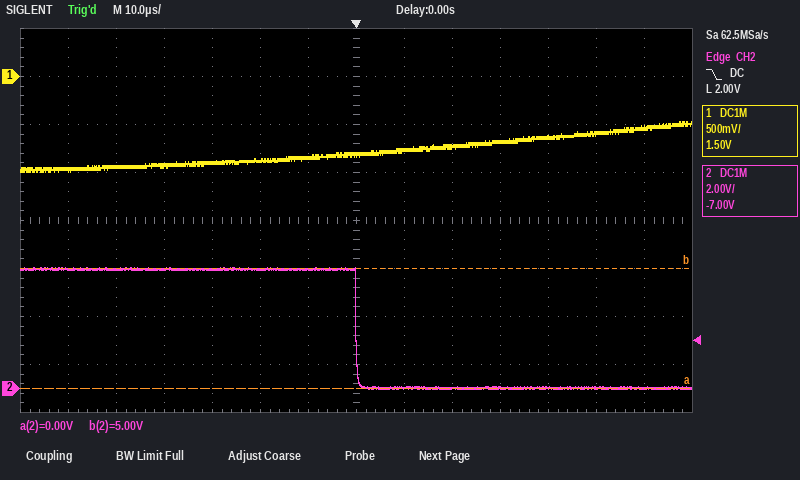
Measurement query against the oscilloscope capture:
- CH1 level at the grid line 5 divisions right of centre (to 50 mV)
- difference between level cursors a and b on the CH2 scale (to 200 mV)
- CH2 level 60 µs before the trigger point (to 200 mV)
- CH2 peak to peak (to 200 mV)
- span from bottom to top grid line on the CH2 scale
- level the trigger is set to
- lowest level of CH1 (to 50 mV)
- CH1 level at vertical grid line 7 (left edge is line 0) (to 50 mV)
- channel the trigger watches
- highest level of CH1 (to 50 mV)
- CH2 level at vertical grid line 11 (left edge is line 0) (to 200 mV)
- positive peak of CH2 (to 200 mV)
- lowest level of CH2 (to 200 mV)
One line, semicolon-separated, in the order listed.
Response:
-600 mV; 5.0 V; 5.0 V; 5.0 V; 16 V; 2.00 V; -1.00 V; -800 mV; CH2; -450 mV; 0.0 V; 5.0 V; 0.0 V
